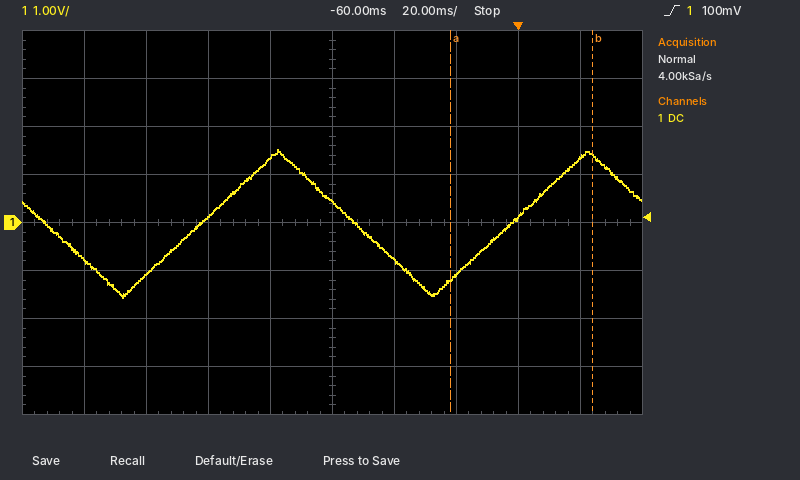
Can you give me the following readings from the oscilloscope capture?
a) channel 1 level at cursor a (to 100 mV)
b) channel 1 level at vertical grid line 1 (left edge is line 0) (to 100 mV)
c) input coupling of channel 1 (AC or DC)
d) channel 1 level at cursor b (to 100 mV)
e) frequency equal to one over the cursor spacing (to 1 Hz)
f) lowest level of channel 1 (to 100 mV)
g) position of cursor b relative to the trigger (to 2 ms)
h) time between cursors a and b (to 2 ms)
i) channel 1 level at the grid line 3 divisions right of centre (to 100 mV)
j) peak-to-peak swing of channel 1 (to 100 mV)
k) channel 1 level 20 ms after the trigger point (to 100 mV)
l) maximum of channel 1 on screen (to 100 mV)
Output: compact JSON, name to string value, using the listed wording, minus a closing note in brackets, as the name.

{"channel 1 level at cursor a": "-1.2 V", "channel 1 level at vertical grid line 1 (left edge is line 0)": "-800 mV", "input coupling of channel 1": "DC", "channel 1 level at cursor b": "1.4 V", "frequency equal to one over the cursor spacing": "22 Hz", "lowest level of channel 1": "-1.6 V", "position of cursor b relative to the trigger": "+24 ms", "time between cursors a and b": "46 ms", "channel 1 level at the grid line 3 divisions right of centre": "100 mV", "peak-to-peak swing of channel 1": "3.1 V", "channel 1 level 20 ms after the trigger point": "1.3 V", "maximum of channel 1 on screen": "1.5 V"}
